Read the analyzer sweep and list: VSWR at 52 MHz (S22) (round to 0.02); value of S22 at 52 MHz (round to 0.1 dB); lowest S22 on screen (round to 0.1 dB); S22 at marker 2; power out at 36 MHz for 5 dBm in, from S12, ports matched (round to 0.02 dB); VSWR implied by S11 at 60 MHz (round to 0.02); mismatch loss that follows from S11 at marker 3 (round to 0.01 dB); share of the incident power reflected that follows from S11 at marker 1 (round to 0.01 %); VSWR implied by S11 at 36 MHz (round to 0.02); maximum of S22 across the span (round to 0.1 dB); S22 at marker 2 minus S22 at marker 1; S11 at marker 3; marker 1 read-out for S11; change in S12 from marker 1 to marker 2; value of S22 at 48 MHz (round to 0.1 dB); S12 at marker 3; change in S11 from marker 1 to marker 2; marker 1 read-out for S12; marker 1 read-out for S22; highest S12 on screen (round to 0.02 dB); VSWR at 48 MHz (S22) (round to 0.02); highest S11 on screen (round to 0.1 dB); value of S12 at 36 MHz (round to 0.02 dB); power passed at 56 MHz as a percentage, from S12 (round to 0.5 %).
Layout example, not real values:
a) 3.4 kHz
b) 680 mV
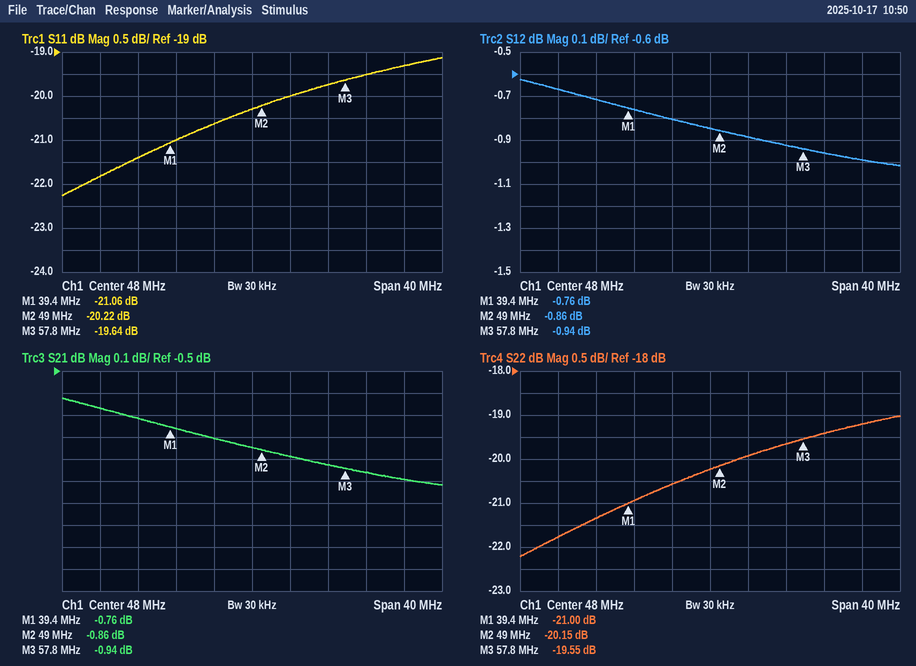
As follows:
a) 1.22
b) -19.9 dB
c) -22.2 dB
d) -20.15 dB
e) 4.28 dBm
f) 1.24
g) 0.05 dB
h) 0.78 %
i) 1.18
j) -19.0 dB
k) 0.85 dB
l) -19.64 dB
m) -21.06 dB
n) -0.10 dB
o) -20.2 dB
p) -0.94 dB
q) 0.84 dB
r) -0.76 dB
s) -21.00 dB
t) -0.62 dB
u) 1.22
v) -19.1 dB
w) -0.72 dB
x) 81.0 %
